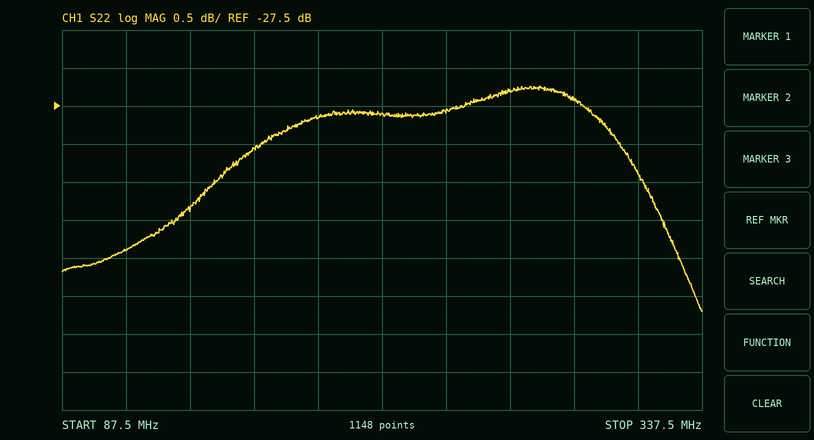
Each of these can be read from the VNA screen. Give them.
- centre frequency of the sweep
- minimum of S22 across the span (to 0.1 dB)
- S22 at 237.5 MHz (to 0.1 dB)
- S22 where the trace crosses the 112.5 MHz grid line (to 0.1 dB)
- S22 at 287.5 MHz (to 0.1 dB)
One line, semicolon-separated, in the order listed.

212.5 MHz; -30.2 dB; -27.6 dB; -29.4 dB; -27.4 dB
